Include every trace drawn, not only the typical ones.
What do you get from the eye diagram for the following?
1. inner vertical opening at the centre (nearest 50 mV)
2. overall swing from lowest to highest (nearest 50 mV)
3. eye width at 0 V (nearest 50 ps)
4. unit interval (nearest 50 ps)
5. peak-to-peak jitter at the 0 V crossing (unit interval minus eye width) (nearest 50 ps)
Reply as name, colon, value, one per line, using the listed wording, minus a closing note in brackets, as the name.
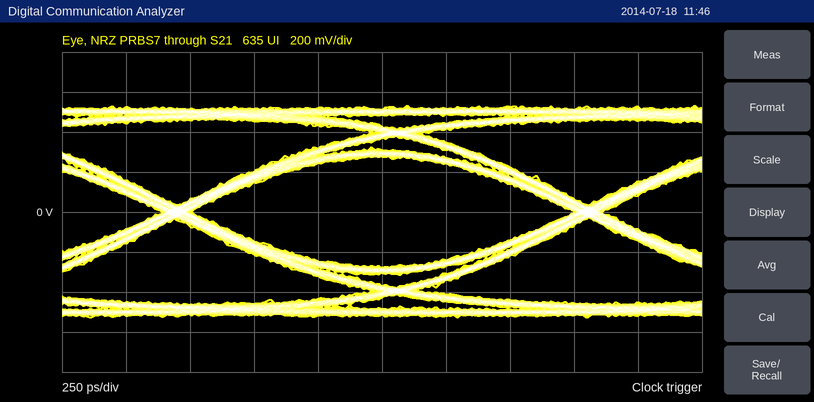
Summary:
inner vertical opening at the centre: 550 mV
overall swing from lowest to highest: 1.05 V
eye width at 0 V: 1.50 ns
unit interval: 1.60 ns
peak-to-peak jitter at the 0 V crossing (unit interval minus eye width): 100 ps
